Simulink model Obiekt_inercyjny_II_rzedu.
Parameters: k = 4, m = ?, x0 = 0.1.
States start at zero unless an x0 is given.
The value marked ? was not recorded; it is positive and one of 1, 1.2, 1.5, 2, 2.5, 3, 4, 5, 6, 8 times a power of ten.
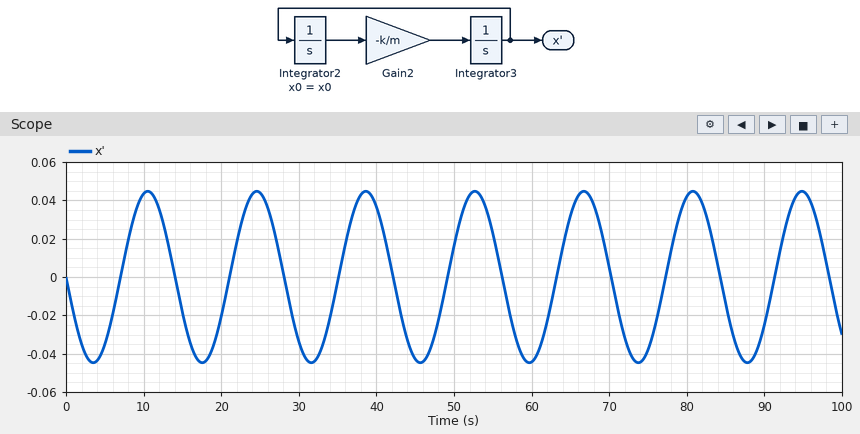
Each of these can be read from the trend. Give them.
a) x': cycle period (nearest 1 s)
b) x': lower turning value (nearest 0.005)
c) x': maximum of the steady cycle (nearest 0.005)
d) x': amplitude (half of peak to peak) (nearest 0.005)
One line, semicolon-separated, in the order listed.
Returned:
14 s; -0.045; 0.045; 0.045
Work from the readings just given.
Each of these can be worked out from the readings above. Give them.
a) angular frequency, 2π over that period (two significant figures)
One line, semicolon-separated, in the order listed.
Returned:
0.45 rad/s
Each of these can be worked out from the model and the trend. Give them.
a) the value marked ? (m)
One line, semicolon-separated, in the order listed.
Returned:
20
